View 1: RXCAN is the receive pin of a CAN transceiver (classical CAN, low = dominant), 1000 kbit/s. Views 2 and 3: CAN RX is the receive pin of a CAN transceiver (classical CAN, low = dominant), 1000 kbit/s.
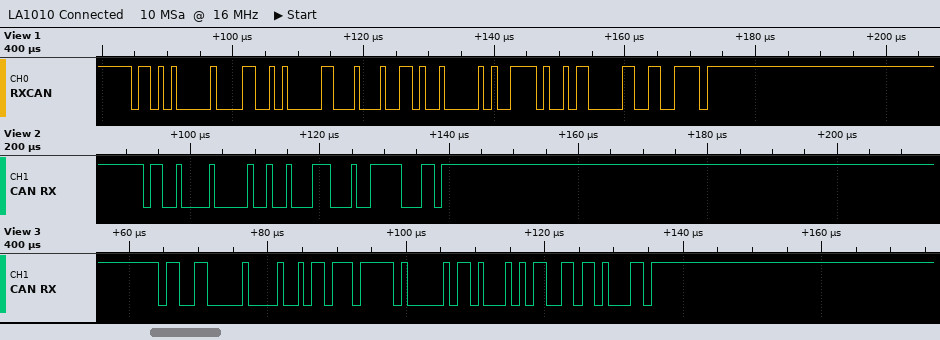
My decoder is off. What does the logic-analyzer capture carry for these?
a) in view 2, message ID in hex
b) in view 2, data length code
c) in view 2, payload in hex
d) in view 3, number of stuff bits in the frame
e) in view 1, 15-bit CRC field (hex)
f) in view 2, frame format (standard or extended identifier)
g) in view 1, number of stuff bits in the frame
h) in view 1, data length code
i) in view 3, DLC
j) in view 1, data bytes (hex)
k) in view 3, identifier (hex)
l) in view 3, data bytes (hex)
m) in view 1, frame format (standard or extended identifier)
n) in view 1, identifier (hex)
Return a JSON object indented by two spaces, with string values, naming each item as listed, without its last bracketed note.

{
  "in view 2, message ID in hex": "0x642",
  "in view 2, data length code": "1",
  "in view 2, payload in hex": "23",
  "in view 3, number of stuff bits in the frame": "3",
  "in view 1, 15-bit CRC field": "0x0267",
  "in view 2, frame format": "standard",
  "in view 1, number of stuff bits in the frame": "4",
  "in view 1, data length code": "6",
  "in view 3, DLC": "4",
  "in view 1, data bytes": "50 44 4D 20 4F 4B",
  "in view 3, identifier": "0x660",
  "in view 3, data bytes": "B7 7E 06 8A",
  "in view 1, frame format": "standard",
  "in view 1, identifier": "0x6A0"
}
